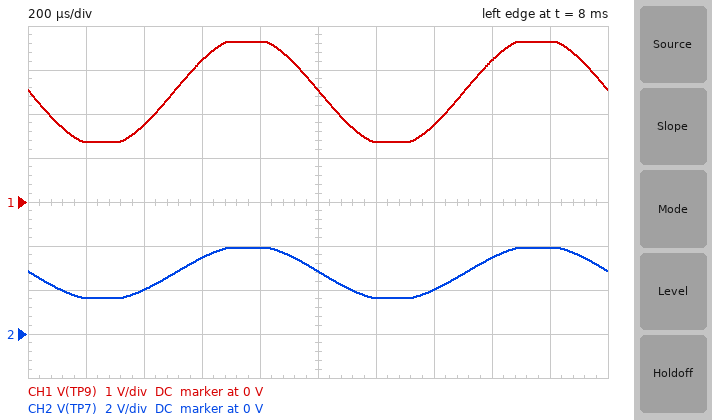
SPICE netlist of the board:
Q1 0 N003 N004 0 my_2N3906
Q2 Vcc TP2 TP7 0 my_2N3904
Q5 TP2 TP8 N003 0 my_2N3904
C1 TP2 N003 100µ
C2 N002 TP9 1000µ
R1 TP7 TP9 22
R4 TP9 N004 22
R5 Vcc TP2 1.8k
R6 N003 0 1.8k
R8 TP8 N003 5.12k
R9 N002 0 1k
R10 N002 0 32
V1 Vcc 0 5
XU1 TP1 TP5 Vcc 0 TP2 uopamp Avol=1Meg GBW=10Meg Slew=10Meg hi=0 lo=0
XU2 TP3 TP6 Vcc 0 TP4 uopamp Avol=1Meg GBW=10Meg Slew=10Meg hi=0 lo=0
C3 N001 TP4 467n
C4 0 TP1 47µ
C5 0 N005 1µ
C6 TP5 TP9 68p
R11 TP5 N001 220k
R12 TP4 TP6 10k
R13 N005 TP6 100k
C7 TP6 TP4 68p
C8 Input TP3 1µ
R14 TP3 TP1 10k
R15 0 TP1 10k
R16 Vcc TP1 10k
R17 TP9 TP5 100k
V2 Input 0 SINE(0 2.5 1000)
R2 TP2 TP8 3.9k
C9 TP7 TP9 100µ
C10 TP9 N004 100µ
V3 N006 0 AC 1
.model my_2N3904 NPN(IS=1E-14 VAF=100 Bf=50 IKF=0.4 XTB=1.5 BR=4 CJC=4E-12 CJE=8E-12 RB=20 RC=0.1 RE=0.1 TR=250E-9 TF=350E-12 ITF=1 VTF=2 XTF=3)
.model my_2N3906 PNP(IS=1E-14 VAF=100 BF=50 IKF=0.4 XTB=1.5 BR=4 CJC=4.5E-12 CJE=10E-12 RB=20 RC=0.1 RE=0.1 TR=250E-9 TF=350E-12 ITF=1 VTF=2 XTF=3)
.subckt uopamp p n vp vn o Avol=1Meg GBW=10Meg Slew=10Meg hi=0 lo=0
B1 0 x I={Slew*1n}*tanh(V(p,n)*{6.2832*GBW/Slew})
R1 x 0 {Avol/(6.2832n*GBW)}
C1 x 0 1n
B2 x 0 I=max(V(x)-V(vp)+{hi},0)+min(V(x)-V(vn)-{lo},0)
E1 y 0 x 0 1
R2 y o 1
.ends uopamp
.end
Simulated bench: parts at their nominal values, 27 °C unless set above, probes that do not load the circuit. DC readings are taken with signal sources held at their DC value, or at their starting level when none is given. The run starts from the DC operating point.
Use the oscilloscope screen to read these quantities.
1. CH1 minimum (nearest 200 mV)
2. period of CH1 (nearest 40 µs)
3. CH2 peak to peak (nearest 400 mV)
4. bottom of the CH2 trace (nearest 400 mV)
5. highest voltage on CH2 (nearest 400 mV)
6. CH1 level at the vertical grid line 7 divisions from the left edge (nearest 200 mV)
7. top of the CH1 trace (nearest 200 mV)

1.4 V
1.00 ms
2.4 V
1.6 V
4.0 V
1.8 V
3.6 V
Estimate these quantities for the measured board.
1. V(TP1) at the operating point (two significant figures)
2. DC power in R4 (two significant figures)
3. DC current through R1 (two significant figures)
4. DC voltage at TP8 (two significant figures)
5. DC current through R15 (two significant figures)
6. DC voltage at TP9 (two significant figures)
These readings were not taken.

2.5 V
550 nW
160 µA
2.5 V
250 µA
2.5 V
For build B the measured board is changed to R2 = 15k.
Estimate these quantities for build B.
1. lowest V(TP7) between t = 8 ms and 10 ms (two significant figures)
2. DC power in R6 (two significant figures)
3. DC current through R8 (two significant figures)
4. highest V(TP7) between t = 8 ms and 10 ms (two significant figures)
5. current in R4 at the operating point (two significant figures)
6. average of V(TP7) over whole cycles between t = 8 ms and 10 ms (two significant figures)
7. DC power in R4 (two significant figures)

1.8 V
920 µW
120 µA
4.1 V
21 mA
3.0 V
10 mW
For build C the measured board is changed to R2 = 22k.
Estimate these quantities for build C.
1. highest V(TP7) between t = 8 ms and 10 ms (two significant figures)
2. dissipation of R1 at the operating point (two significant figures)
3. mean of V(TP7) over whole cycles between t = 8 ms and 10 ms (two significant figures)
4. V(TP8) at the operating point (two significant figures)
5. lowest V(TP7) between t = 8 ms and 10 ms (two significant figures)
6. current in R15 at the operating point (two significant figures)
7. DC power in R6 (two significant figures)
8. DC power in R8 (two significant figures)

4.2 V
15 mW
3.1 V
1.7 V
1.9 V
250 µA
750 µW
50 µW
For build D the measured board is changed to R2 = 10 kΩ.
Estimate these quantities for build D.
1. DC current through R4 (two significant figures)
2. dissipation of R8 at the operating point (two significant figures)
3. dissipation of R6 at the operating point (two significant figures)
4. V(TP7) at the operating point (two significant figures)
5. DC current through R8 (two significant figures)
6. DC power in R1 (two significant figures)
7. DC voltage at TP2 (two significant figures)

12 mA
79 µW
1.3 mW
2.8 V
120 µA
3.1 mW
3.5 V
